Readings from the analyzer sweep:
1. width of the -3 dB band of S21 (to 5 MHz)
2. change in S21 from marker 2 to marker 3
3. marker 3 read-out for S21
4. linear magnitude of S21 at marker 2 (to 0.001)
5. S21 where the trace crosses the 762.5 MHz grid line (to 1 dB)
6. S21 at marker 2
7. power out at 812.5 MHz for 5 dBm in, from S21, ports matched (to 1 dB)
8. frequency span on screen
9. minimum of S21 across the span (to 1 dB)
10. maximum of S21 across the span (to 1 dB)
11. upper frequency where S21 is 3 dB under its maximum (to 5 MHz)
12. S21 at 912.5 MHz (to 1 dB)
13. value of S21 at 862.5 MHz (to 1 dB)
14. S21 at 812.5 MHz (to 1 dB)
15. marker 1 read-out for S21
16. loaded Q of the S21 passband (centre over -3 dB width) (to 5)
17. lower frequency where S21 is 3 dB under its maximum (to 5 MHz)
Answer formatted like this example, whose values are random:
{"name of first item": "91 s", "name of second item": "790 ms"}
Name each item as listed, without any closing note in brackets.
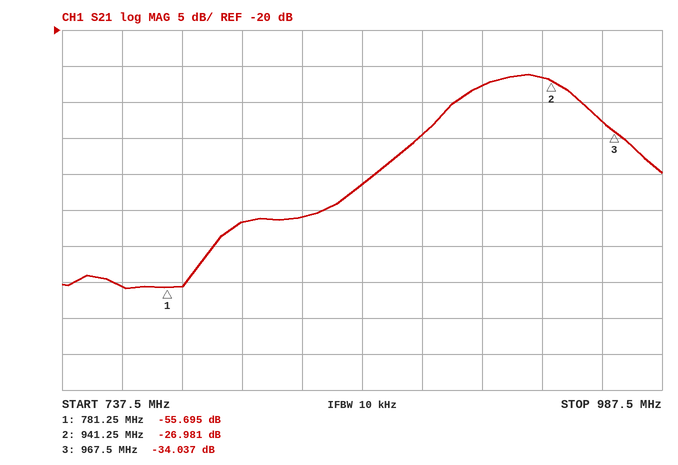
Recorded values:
{"width of the -3 dB band of S21": "45 MHz", "change in S21 from marker 2 to marker 3": "-7.056 dB", "marker 3 read-out for S21": "-34.037 dB", "linear magnitude of S21 at marker 2": "0.045", "S21 where the trace crosses the 762.5 MHz grid line": "-56 dB", "S21 at marker 2": "-26.981 dB", "power out at 812.5 MHz for 5 dBm in, from S21, ports matched": "-42 dBm", "frequency span on screen": "250 MHz", "minimum of S21 across the span": "-56 dB", "maximum of S21 across the span": "-26 dB", "upper frequency where S21 is 3 dB under its maximum": "950 MHz", "S21 at 912.5 MHz": "-28 dB", "value of S21 at 862.5 MHz": "-41 dB", "S21 at 812.5 MHz": "-47 dB", "marker 1 read-out for S21": "-55.695 dB", "loaded Q of the S21 passband (centre over -3 dB width)": "20", "lower frequency where S21 is 3 dB under its maximum": "905 MHz"}
